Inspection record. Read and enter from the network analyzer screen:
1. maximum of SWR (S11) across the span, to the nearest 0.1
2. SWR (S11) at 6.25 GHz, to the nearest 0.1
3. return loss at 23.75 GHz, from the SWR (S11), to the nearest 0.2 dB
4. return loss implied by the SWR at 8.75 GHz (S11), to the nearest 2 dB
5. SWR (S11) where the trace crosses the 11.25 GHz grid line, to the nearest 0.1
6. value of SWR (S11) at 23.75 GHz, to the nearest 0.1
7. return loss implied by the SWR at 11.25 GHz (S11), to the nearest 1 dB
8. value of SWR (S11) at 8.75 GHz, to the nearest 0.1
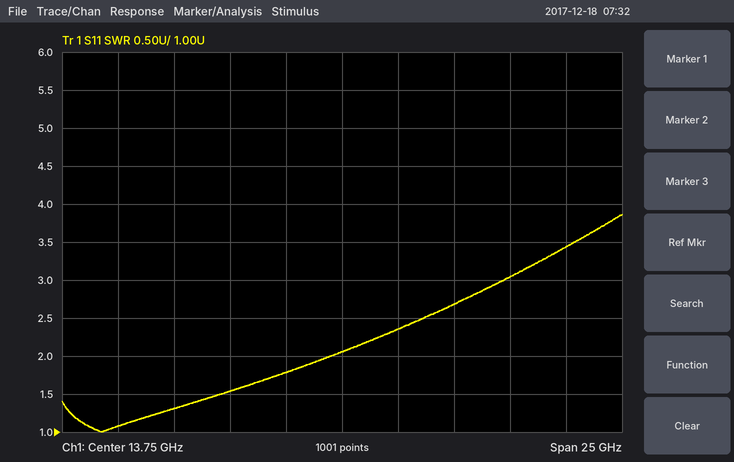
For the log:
3.9
1.3
5.2 dB
14 dB
1.8
3.4
11 dB
1.5
